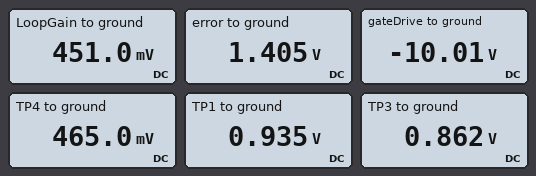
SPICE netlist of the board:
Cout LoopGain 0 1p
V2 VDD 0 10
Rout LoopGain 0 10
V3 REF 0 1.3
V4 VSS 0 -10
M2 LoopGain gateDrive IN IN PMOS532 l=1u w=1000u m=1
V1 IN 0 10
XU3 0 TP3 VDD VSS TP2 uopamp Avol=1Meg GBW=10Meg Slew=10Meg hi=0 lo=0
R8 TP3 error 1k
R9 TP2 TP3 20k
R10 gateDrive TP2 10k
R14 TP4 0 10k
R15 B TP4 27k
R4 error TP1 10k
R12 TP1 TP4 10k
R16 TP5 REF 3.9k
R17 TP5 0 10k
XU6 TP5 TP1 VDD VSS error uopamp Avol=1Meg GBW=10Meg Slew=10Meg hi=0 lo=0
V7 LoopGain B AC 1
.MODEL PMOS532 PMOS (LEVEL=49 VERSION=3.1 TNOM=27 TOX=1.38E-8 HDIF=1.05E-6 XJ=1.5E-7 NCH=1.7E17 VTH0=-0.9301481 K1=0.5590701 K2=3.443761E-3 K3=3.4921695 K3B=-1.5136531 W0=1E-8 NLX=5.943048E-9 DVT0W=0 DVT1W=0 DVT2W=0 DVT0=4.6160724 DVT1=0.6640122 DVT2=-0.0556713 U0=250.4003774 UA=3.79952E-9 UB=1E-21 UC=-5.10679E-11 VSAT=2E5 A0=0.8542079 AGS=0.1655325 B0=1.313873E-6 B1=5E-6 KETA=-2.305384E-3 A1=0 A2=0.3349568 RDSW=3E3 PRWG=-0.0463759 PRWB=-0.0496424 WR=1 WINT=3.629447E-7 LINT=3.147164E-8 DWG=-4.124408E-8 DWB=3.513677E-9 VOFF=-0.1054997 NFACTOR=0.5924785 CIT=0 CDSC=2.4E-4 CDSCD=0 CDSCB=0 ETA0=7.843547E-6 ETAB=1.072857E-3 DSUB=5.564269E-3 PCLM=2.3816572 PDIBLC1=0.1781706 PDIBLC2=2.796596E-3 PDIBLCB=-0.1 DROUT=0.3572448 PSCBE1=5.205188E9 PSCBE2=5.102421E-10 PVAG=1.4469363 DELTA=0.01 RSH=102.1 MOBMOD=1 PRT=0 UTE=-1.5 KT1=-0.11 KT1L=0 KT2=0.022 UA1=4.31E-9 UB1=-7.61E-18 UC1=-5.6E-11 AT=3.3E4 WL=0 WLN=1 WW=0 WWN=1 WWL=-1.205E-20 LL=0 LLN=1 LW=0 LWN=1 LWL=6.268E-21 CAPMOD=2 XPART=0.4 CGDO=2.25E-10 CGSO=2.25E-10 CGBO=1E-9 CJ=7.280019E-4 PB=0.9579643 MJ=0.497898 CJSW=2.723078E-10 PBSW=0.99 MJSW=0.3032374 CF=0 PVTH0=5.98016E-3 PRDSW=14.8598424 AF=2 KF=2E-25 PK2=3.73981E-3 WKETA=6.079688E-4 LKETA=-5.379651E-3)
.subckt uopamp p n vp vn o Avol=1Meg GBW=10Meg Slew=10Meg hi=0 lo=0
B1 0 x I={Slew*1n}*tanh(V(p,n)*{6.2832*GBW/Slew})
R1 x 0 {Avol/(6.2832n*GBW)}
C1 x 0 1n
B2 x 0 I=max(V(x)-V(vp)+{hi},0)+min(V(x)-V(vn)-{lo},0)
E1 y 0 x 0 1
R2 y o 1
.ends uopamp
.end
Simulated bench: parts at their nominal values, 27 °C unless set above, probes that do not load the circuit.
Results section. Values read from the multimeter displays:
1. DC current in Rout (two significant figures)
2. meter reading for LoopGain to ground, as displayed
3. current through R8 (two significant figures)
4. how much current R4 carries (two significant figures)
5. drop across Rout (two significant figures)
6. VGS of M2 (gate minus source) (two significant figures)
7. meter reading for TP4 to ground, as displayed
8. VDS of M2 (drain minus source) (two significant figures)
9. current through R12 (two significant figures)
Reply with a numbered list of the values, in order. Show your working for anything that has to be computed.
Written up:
1. (451 mV) / 10 Ω = 45 mA
2. 451.0 mV
3. (1.405 V - 862 mV) / 1 kΩ = 540 µA
4. (1.405 V - 935 mV) / 10 kΩ = 47 µA
5. 451 mV = 450 mV
6. -10.01 V - 10 V = -20 V
7. 465.0 mV
8. 451 mV - 10 V = -9.5 V
9. (935 mV - 465 mV) / 10 kΩ = 47 µA
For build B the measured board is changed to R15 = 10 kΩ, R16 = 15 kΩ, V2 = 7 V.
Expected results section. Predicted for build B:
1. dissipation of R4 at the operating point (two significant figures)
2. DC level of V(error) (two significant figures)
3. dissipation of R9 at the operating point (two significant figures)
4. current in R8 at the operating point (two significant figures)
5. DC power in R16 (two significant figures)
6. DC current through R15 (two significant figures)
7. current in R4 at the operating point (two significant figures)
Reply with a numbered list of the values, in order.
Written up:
1. 3.9 µW
2. 720 mV
3. 5.2 mW
4. 510 µA
5. 41 µW
6. 13 µA
7. 20 µA
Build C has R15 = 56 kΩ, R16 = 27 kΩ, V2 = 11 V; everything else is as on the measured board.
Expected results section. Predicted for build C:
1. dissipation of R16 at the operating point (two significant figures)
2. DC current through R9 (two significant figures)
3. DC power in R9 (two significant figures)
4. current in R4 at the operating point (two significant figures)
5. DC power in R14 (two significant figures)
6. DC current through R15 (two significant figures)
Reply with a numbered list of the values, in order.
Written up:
1. 33 µW
2. 500 µA
3. 5.0 mW
4. 15 µA
5. 3.9 µW
6. 4.5 µA
